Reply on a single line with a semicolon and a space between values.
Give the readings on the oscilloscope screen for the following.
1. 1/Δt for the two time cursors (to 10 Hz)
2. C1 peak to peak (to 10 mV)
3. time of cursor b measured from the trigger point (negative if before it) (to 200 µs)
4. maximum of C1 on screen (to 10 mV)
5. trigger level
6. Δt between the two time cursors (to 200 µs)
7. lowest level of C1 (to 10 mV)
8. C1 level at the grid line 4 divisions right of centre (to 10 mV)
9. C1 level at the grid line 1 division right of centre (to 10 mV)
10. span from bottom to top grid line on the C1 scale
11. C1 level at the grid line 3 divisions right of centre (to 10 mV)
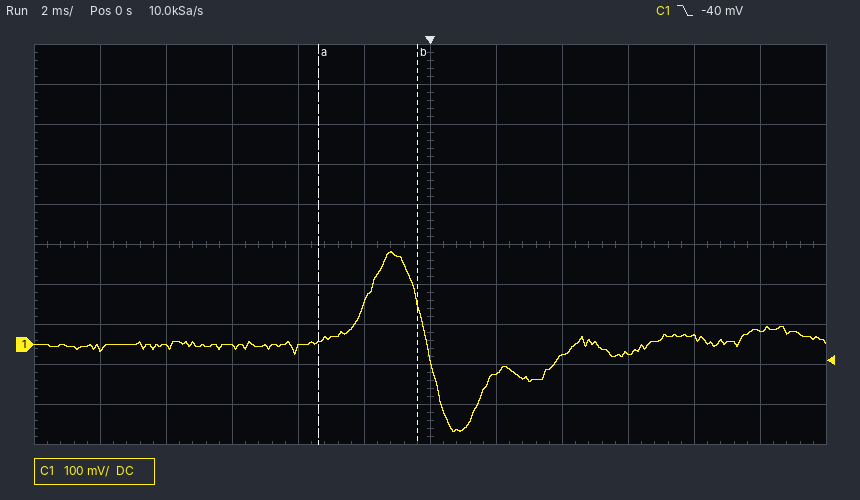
330 Hz; 450 mV; -400 µs; 230 mV; -40 mV; 3.0 ms; -220 mV; 20 mV; -70 mV; 1 V; -20 mV
